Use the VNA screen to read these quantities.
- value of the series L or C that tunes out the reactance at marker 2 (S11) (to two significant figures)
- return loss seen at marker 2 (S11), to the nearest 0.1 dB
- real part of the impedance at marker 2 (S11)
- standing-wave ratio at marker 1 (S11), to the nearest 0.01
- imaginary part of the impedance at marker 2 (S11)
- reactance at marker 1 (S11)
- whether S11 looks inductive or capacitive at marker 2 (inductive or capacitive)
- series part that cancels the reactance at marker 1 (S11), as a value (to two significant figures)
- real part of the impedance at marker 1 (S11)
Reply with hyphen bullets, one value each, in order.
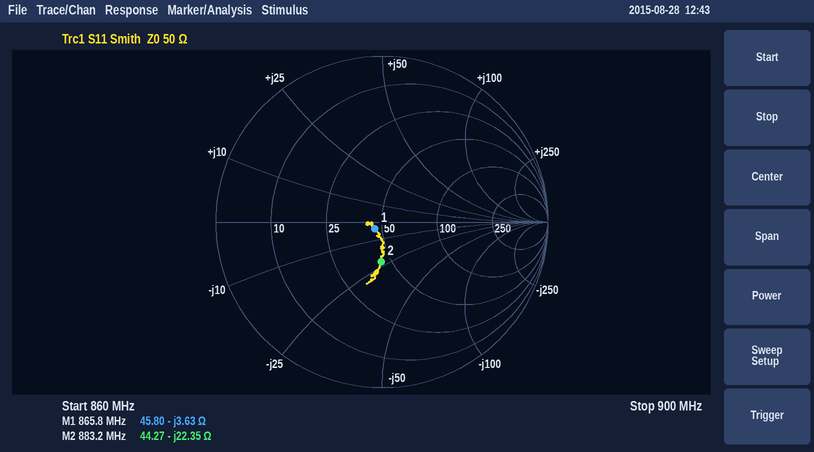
- 4.0 nH
- 12.5 dB
- 44.27 Ω
- 1.12
- -22.35 Ω
- -3.63 Ω
- capacitive
- 670 pH
- 45.80 Ω
